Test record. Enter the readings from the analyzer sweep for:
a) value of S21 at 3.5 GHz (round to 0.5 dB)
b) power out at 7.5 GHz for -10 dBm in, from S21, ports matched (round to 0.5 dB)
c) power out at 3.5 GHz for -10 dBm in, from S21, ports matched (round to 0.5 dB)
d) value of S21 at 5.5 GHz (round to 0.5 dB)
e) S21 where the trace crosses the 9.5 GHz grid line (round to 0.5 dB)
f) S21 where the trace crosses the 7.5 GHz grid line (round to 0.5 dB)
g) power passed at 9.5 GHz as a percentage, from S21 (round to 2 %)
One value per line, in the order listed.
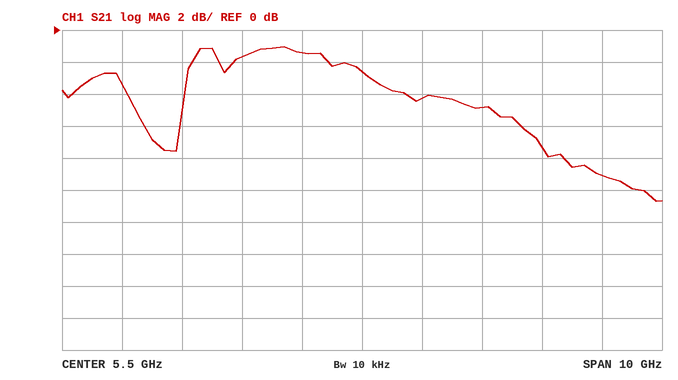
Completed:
-1.5 dB
-15.0 dBm
-11.5 dBm
-2.5 dB
-9.0 dB
-5.0 dB
12 %
